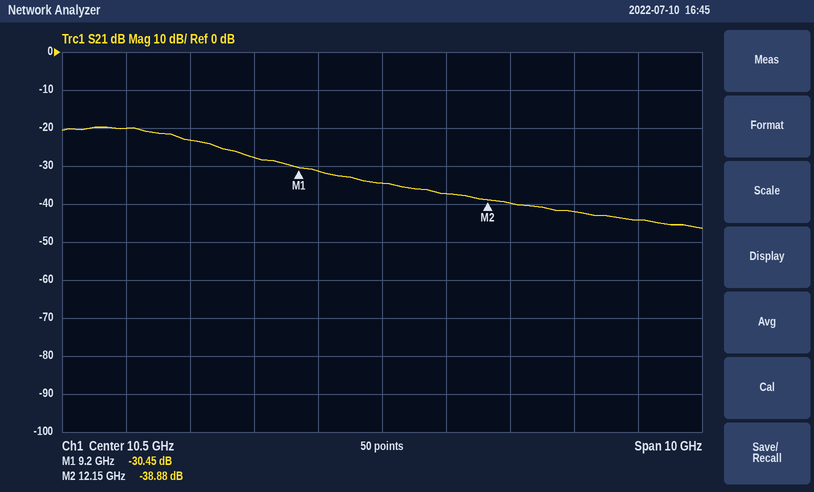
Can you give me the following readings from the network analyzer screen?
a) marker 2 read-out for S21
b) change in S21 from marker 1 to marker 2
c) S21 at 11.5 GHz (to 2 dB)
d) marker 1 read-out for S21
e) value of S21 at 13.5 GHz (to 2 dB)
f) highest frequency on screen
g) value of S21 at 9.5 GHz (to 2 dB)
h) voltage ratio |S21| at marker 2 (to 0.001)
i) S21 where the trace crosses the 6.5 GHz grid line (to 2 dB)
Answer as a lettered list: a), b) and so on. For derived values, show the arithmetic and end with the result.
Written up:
a) -38.88 dB
b) -38.88 − (-30.45) = -8.43 dB
c) -38 dB
d) -30.45 dB
e) -42 dB
f) 15.5 GHz
g) -32 dB
h) 10^(-38.88/20) ≈ 0.011
i) -20 dB
